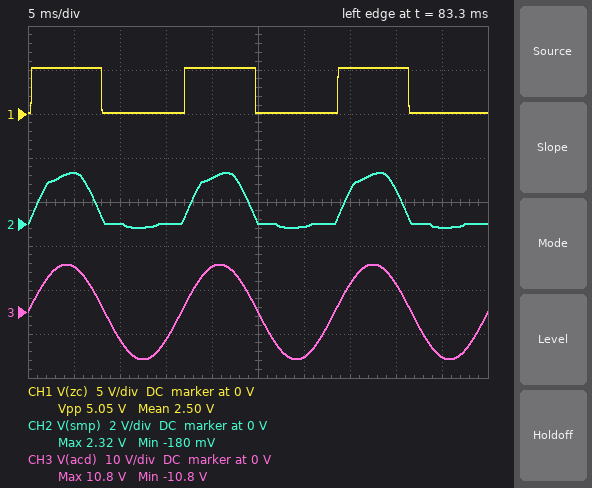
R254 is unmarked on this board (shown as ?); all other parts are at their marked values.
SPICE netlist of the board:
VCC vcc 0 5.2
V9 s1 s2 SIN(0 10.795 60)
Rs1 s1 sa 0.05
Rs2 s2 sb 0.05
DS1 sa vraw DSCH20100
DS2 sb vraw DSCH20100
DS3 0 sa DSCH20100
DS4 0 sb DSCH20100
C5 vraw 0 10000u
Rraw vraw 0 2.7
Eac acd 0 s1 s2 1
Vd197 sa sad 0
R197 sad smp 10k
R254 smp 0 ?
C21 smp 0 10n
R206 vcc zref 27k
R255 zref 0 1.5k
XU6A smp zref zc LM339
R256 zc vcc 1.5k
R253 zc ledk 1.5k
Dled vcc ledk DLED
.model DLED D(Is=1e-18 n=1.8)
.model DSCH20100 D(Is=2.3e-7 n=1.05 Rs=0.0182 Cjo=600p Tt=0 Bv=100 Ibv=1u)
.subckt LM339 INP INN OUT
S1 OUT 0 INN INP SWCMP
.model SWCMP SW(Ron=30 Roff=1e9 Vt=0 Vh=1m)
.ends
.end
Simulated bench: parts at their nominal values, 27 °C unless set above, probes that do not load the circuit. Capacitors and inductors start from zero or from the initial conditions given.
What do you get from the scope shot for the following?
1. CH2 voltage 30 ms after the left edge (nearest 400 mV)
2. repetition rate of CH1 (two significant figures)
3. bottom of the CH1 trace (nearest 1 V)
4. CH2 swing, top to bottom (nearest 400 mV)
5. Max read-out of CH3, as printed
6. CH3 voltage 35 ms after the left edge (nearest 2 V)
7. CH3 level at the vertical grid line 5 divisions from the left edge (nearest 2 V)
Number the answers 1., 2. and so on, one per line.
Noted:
1. 0 V
2. 60 Hz
3. 0 V
4. 2.4 V
5. 10.8 V
6. 6 V
7. 0 V
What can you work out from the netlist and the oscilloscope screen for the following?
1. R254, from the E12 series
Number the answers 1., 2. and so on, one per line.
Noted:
1. 3.3 kΩ
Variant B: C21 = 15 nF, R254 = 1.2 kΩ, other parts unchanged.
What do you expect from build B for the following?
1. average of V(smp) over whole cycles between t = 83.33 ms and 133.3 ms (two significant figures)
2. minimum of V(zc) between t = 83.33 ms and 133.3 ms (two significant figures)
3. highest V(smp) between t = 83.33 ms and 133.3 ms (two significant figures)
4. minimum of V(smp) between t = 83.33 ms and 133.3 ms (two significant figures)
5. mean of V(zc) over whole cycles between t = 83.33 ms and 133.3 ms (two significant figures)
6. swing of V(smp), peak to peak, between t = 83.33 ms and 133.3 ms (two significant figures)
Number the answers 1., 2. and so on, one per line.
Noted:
1. 320 mV
2. 170 mV
3. 1.0 V
4. -75 mV
5. 2.3 V
6. 1.1 V
